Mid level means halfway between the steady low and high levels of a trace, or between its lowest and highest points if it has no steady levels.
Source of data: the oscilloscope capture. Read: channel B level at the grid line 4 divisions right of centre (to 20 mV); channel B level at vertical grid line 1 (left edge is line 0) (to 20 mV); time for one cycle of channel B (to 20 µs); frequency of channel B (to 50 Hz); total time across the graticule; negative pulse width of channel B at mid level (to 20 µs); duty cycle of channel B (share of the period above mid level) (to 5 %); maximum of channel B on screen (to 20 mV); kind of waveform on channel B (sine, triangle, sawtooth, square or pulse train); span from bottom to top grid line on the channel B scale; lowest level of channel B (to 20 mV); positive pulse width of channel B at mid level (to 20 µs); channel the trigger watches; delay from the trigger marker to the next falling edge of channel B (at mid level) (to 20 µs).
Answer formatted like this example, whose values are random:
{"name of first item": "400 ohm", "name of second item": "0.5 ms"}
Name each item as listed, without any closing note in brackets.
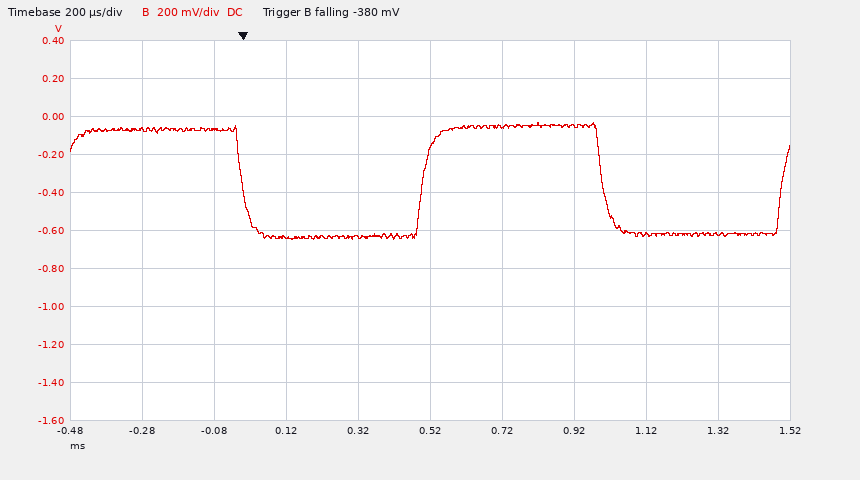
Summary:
{"channel B level at the grid line 4 divisions right of centre": "-620 mV", "channel B level at vertical grid line 1 (left edge is line 0)": "-60 mV", "time for one cycle of channel B": "1.00 ms", "frequency of channel B": "1.00 kHz", "total time across the graticule": "2 ms", "negative pulse width of channel B at mid level": "500 µs", "duty cycle of channel B (share of the period above mid level)": "50 %", "maximum of channel B on screen": "-40 mV", "kind of waveform on channel B": "square", "span from bottom to top grid line on the channel B scale": "2 V", "lowest level of channel B": "-640 mV", "positive pulse width of channel B at mid level": "500 µs", "channel the trigger watches": "channel B", "delay from the trigger marker to the next falling edge of channel B (at mid level)": "1.00 ms"}
